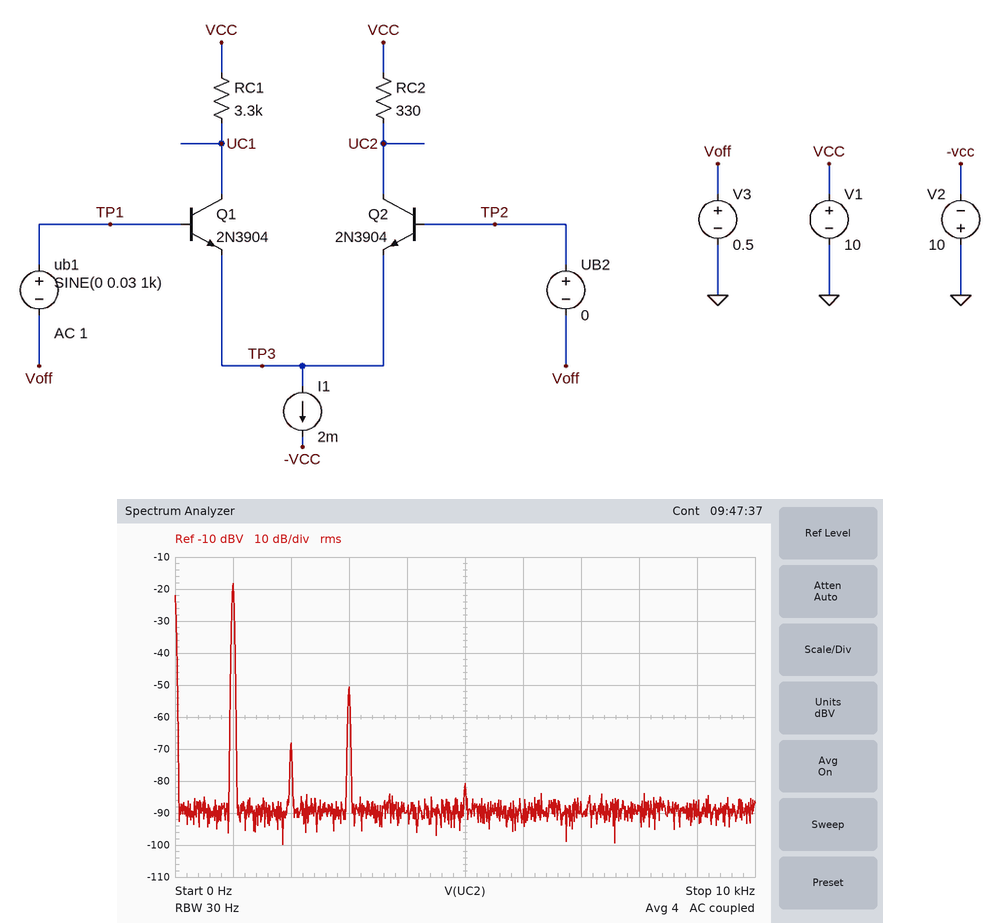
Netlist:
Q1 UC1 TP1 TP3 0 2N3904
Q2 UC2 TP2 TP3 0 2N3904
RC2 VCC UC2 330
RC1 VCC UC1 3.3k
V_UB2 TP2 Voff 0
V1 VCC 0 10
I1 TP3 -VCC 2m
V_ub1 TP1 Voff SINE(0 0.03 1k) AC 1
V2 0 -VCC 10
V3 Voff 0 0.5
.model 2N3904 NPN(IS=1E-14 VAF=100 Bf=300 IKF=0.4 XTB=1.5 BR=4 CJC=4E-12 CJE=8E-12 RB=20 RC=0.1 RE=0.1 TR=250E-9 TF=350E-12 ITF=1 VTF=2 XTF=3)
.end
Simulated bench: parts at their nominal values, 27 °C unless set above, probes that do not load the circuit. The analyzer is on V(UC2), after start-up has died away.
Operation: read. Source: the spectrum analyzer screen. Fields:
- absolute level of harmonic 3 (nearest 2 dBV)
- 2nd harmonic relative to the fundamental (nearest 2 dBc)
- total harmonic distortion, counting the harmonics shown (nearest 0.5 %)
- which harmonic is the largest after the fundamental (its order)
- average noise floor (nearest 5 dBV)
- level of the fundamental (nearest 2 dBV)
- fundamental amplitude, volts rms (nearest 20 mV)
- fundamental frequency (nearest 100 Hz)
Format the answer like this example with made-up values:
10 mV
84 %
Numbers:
-50 dBV
-50 dBc
2.5 %
3
-90 dBV
-18 dBV
120 mV
1.0 kHz
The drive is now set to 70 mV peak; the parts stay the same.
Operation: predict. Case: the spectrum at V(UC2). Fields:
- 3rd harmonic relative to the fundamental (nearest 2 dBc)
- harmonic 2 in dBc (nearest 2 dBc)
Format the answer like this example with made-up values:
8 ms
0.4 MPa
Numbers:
-20 dBc
-46 dBc
